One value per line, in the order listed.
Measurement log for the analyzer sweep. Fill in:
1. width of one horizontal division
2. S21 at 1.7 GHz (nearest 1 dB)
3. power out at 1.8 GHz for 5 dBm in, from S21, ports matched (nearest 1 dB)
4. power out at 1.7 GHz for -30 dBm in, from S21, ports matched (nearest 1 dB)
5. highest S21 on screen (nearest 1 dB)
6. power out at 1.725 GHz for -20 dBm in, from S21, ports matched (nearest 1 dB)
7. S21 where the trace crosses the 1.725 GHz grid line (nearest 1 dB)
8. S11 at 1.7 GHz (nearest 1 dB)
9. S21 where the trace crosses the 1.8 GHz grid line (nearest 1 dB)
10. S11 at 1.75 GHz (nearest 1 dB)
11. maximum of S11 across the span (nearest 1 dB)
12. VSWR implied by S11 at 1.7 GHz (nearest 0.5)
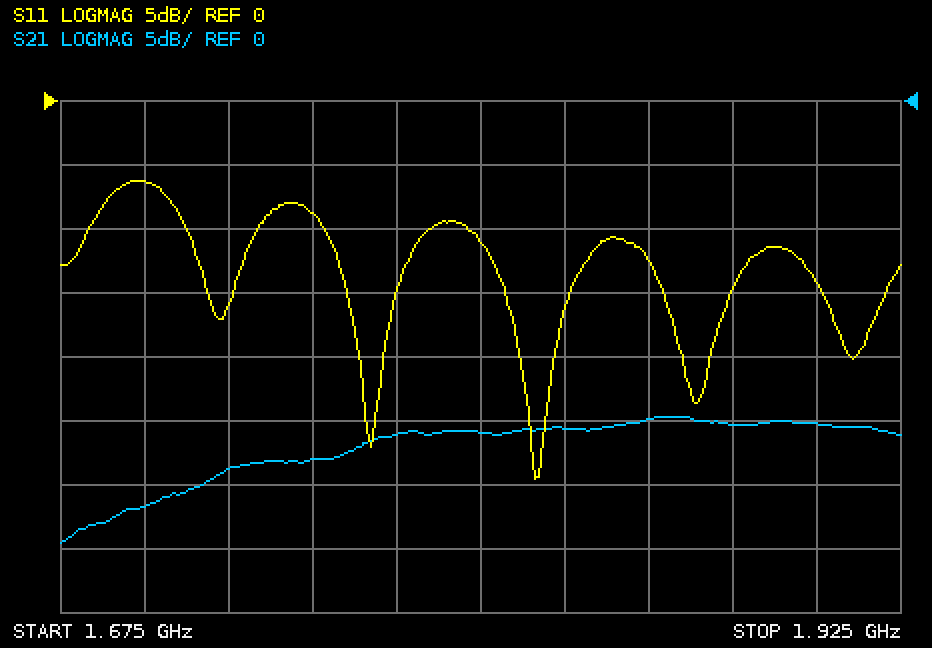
25 MHz
-32 dB
-21 dBm
-62 dBm
-25 dB
-49 dBm
-29 dB
-6 dB
-26 dB
-9 dB
-6 dB
3.0
